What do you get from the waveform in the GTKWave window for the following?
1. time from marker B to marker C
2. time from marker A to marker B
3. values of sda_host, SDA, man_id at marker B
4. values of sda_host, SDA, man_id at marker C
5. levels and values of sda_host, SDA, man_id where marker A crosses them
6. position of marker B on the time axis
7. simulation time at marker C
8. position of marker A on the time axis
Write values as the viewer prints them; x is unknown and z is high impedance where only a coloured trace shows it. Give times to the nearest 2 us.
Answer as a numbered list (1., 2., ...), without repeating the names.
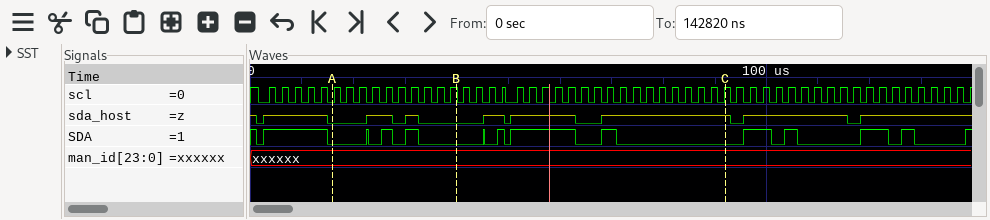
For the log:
1. 52 us
2. 24 us
3. sda_host=0, SDA=0, man_id=xxxxxx
4. sda_host=z, SDA=0, man_id=xxxxxx
5. sda_host=0, SDA=0, man_id=xxxxxx
6. 40 us
7. 92 us
8. 16 us
